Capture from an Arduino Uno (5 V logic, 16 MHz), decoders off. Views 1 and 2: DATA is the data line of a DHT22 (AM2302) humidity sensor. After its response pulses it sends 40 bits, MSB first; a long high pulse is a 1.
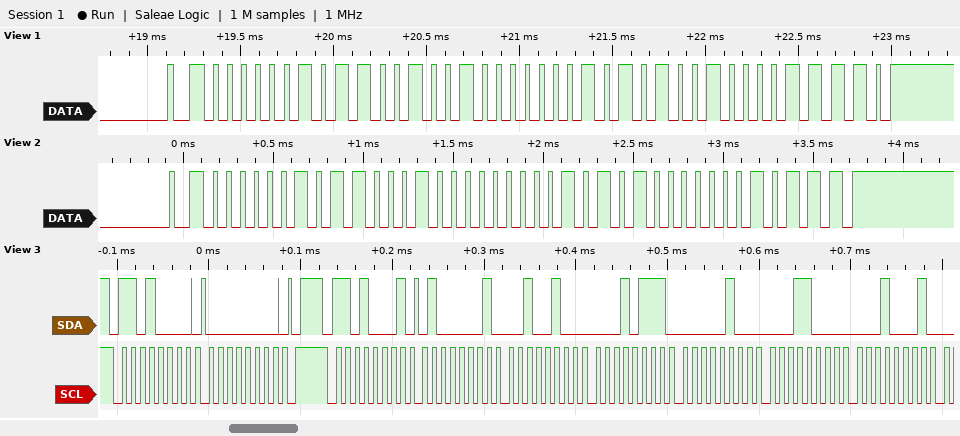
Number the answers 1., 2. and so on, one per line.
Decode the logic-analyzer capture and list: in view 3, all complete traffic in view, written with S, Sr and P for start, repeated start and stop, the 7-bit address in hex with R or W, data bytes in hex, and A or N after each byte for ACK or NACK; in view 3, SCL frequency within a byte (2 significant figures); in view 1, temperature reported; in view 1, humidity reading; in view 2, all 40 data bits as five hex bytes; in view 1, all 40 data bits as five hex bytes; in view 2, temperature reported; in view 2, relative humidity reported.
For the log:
1. S 68W A 00 A P S 68R A 41 A 24 A 17 A 04 A 18 A 11 A
2. 100 kHz
3. 33.8 °C
4. 71.3 %
5. 02 C4 01 50 17
6. 02 C9 01 52 1E
7. 33.6 °C
8. 70.8 %
